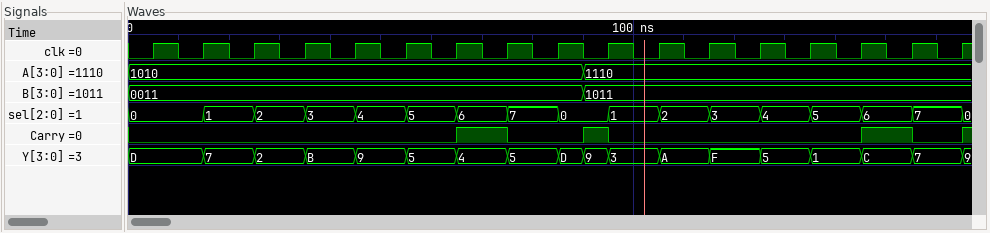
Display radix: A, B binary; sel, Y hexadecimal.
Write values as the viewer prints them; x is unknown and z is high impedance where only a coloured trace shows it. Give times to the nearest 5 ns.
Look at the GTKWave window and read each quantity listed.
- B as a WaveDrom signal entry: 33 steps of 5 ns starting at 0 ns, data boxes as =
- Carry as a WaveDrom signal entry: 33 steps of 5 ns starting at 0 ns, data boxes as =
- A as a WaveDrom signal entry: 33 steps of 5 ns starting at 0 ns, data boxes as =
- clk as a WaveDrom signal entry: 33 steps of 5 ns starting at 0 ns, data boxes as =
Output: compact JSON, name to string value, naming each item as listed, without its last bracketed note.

{"B as a WaveDrom signal entry: 33 steps of 5 ns starting at 0 ns, data boxes as =": "{name: 'B', wave: '=.................=..............', data: '0011 1011'}", "Carry as a WaveDrom signal entry: 33 steps of 5 ns starting at 0 ns, data boxes as =": "{name: 'Carry', wave: '0............1.0..10.........1.0.'}", "A as a WaveDrom signal entry: 33 steps of 5 ns starting at 0 ns, data boxes as =": "{name: 'A', wave: '=.................=..............', data: '1010 1110'}", "clk as a WaveDrom signal entry: 33 steps of 5 ns starting at 0 ns, data boxes as =": "{name: 'clk', wave: '010101010101010101010101010101010'}"}
